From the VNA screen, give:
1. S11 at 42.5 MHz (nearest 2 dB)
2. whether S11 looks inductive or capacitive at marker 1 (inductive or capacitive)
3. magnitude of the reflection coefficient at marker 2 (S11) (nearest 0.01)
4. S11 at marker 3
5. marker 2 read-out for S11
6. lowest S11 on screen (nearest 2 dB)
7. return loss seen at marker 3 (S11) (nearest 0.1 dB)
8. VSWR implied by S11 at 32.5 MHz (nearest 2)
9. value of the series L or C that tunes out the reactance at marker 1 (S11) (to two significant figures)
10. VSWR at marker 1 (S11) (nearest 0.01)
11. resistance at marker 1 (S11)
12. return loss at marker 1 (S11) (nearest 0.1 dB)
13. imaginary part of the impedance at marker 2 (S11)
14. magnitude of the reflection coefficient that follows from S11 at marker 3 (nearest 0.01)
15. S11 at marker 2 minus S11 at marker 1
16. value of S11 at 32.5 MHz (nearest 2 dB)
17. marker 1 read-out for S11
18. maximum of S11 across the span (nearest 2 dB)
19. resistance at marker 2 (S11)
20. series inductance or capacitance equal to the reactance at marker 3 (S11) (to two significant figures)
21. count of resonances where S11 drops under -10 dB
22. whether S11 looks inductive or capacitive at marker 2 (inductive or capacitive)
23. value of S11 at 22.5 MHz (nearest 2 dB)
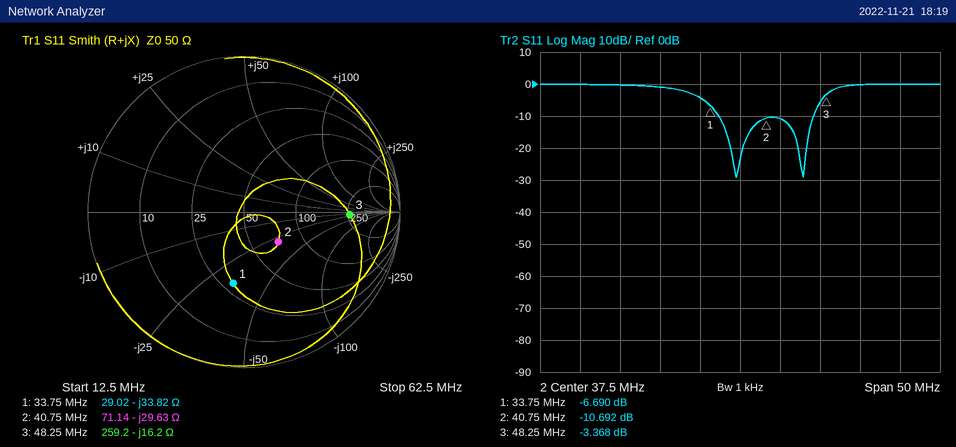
-10 dB
capacitive
0.29
-3.368 dB
-10.692 dB
-30 dB
3.4 dB
4
160 nH
2.72
29.02 Ω
6.7 dB
-29.63 Ω
0.68
-4.002 dB
-4 dB
-6.690 dB
0 dB
71.14 Ω
200 pF
2
capacitive
0 dB
